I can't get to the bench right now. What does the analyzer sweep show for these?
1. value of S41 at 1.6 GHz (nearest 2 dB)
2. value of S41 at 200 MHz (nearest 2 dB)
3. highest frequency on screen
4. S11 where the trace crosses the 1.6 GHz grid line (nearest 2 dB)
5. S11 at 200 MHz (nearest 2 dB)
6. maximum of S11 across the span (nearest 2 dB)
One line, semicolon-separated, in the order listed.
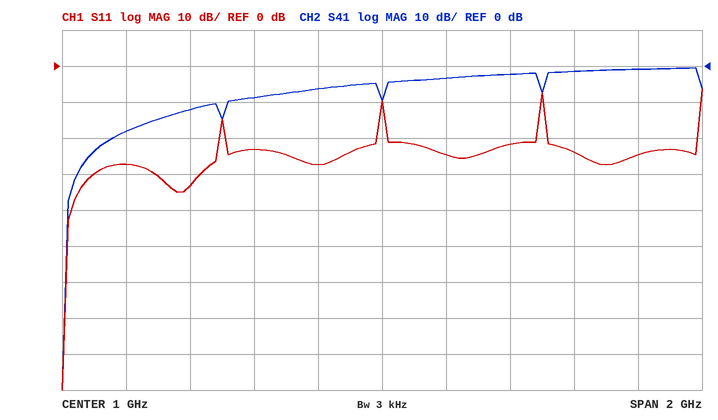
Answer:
-2 dB; -18 dB; 2 GHz; -24 dB; -28 dB; -6 dB
